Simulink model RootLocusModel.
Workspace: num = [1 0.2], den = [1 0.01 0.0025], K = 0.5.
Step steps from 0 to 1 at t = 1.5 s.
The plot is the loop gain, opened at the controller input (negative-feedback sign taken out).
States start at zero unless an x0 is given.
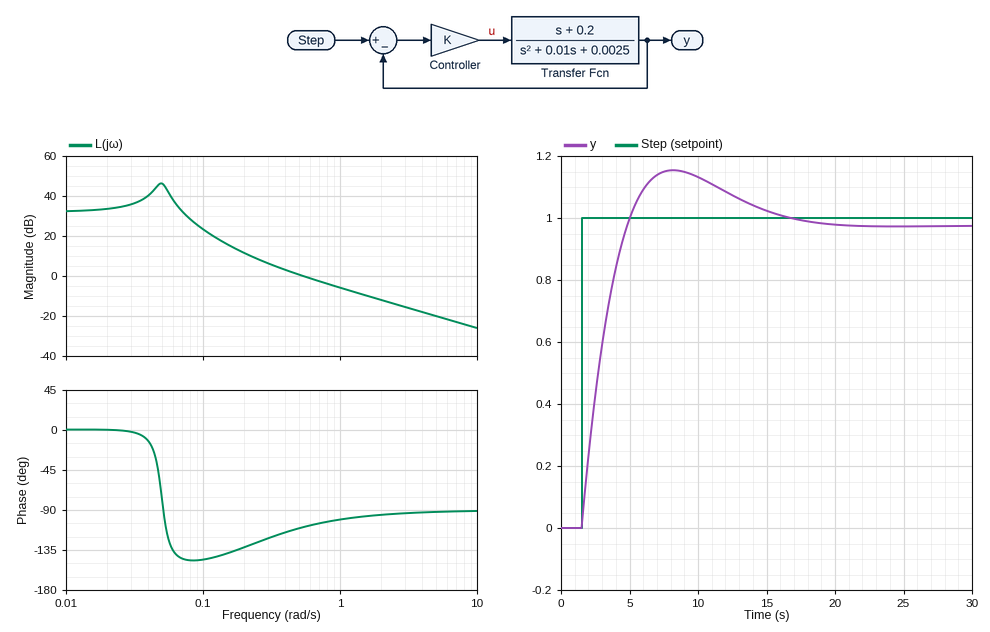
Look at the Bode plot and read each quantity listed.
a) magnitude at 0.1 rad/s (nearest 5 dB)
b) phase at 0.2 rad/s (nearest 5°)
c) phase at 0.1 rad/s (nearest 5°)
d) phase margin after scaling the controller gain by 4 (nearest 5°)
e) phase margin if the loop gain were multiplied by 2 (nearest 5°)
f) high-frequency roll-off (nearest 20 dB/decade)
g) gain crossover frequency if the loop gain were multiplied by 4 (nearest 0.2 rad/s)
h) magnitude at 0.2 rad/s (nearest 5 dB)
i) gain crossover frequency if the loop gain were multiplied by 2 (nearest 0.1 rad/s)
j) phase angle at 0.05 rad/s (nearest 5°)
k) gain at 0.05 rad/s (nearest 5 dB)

25 dB
-130°
-145°
85°
80°
-20 dB/decade
2.0 rad/s
10 dB
1.0 rad/s
-75°
45 dB
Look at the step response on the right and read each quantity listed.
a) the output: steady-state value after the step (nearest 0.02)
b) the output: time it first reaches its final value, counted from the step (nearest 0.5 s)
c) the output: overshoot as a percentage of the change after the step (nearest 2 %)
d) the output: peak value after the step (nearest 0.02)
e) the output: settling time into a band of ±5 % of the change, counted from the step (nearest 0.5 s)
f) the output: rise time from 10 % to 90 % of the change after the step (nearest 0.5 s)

0.98
3.5 s
18 %
1.16
13.5 s
2.5 s
